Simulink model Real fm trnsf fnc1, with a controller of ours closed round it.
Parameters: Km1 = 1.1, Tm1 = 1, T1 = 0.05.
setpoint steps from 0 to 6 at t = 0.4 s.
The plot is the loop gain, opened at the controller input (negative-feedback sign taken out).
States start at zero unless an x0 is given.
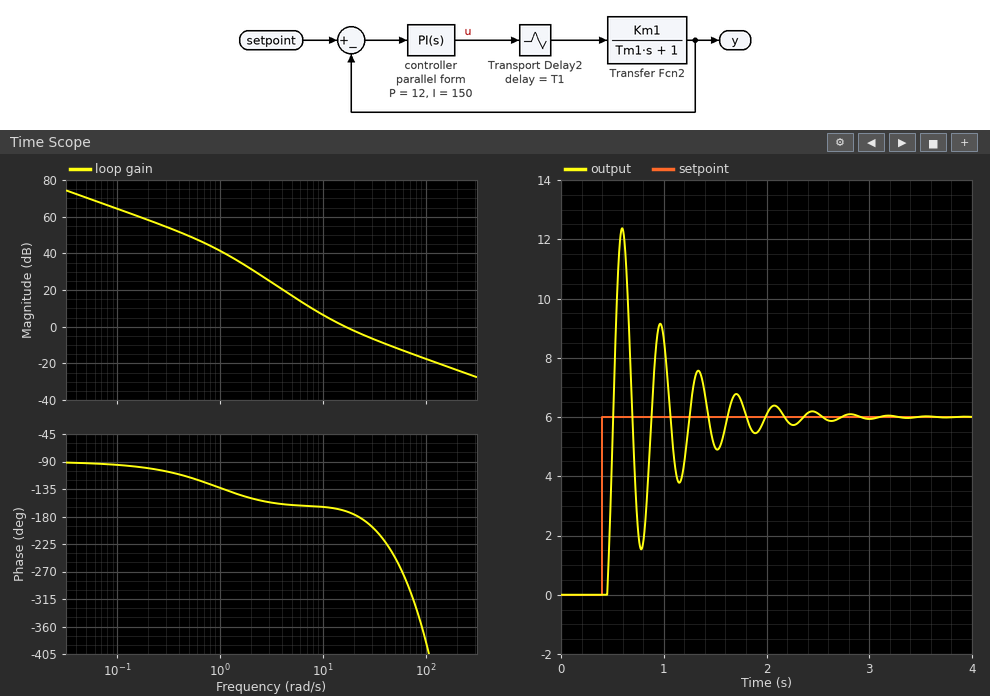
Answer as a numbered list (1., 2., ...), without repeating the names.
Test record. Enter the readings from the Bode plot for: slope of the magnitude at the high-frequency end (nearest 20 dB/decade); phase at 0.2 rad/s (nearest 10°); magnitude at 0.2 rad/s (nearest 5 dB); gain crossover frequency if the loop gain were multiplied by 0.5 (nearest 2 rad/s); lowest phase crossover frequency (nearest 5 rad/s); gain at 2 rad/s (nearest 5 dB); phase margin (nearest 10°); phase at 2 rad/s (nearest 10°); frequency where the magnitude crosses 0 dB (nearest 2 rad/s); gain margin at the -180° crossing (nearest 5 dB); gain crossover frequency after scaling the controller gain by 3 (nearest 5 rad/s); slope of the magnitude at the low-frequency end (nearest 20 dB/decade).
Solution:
1. -20 dB/decade
2. -100°
3. 60 dB
4. 10 rad/s
5. 20 rad/s
6. 30 dB
7. 10°
8. -150°
9. 16 rad/s
10. 5 dB
11. 40 rad/s
12. -20 dB/decade
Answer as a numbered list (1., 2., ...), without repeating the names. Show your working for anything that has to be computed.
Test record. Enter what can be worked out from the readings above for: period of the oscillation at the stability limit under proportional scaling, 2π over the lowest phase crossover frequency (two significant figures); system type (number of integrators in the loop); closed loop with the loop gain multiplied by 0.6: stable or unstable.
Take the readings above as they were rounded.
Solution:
1. 2π / 20 = 0.31 s
2. 1
3. stable
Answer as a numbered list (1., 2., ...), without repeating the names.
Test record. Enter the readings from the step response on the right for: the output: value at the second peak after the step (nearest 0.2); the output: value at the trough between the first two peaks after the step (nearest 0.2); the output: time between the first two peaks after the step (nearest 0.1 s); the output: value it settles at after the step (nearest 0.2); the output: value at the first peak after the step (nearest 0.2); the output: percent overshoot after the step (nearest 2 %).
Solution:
1. 9.2
2. 1.6
3. 0.4 s
4. 6.0
5. 12.4
6. 106 %
